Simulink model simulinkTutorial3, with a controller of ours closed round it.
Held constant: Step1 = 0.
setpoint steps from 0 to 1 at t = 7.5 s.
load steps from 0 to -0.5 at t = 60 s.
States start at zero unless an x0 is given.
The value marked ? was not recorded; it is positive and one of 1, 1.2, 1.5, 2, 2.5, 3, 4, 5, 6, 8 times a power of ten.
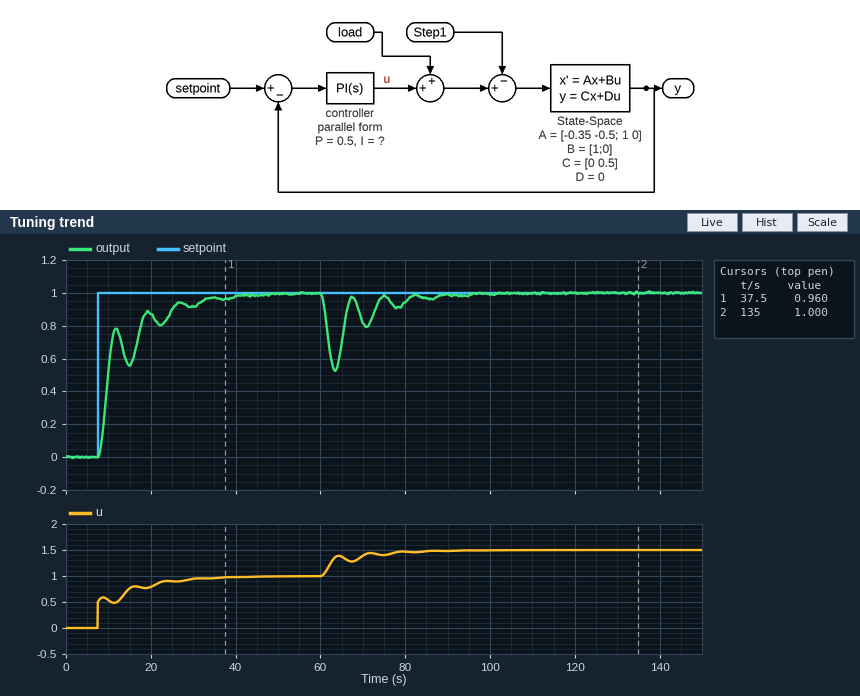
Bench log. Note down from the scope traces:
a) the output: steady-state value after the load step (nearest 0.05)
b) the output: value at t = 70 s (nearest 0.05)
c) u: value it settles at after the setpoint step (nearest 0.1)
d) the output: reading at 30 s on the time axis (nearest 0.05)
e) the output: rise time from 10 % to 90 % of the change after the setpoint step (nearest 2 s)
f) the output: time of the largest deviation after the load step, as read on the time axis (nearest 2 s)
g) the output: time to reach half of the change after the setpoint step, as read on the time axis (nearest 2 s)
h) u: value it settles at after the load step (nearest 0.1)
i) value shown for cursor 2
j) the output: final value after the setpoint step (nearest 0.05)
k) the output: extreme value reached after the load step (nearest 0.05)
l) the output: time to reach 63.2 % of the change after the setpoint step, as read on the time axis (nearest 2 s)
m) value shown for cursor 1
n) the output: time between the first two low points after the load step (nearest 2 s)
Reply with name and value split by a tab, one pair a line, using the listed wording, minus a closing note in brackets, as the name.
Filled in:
the output: steady-state value after the load step	1.00
the output: value at t = 70 s	0.80
u: value it settles at after the setpoint step	1.0
the output: reading at 30 s on the time axis	0.90
the output: rise time from 10 % to 90 % of the change after the setpoint step	16 s
the output: time of the largest deviation after the load step, as read on the time axis	64 s
the output: time to reach half of the change after the setpoint step, as read on the time axis	10 s
u: value it settles at after the load step	1.5
value shown for cursor 2	1.000
the output: final value after the setpoint step	1.00
the output: extreme value reached after the load step	0.55
the output: time to reach 63.2 % of the change after the setpoint step, as read on the time axis	10 s
value shown for cursor 1	0.960
the output: time between the first two low points after the load step	8 s
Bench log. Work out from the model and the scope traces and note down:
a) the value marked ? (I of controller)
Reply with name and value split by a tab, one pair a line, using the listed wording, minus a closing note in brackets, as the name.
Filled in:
the value marked ?	0.15
